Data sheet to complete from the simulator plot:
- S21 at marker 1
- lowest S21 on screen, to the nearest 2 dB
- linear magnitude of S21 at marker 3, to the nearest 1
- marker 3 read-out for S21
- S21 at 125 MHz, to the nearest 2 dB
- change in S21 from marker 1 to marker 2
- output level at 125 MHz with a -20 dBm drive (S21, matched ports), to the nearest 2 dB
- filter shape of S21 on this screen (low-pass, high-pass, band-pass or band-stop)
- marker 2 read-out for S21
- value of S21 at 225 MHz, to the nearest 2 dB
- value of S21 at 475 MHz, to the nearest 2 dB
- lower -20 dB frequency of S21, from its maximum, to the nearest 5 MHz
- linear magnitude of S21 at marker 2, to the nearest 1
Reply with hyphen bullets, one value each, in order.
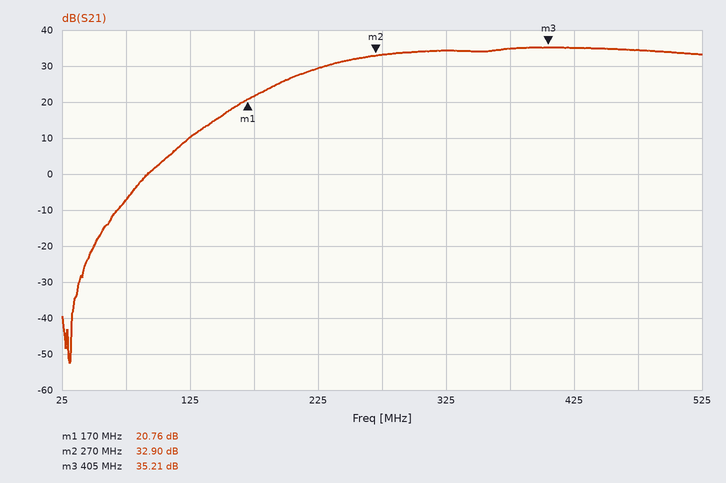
- 20.76 dB
- -52 dB
- 58
- 35.21 dB
- 10 dB
- 12.14 dB
- -10 dBm
- high-pass
- 32.90 dB
- 30 dB
- 34 dB
- 145 MHz
- 44
